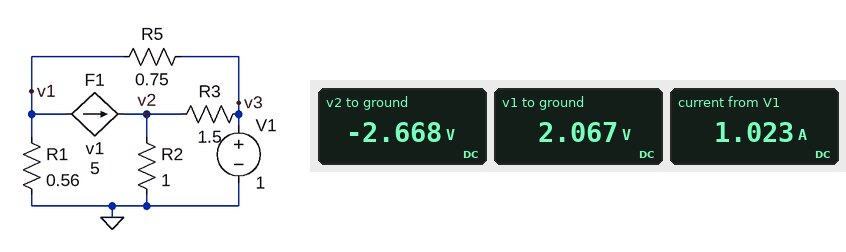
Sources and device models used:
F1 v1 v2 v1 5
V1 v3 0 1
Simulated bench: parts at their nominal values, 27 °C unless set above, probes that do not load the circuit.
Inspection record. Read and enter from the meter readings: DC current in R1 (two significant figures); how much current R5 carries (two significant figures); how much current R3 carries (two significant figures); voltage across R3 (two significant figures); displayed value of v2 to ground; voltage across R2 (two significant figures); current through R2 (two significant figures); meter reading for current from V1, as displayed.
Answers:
3.7 A
1.4 A
2.4 A
3.7 V
-2.668 V
2.7 V
2.7 A
1.023 A
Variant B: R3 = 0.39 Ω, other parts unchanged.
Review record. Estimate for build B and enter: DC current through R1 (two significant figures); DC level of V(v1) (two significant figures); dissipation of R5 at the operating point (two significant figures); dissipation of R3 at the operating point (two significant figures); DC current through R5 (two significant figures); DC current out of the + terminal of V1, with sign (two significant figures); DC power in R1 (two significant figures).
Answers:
8.5 A
-4.7 V
44 W
46 W
7.7 A
-3.2 A
40 W
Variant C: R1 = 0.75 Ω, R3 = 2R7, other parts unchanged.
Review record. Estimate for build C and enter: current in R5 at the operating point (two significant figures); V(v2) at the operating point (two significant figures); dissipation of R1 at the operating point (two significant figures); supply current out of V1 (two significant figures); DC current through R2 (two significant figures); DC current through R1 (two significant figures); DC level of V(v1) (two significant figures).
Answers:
420 mA
-1.3 V
2.3 W
440 mA
1.3 A
1.8 A
1.3 V
